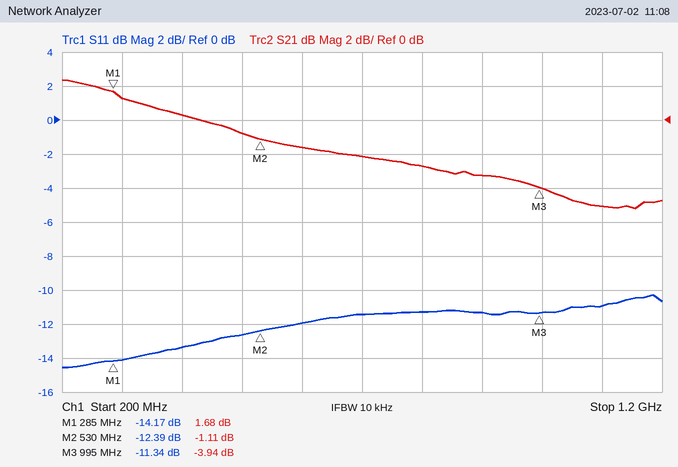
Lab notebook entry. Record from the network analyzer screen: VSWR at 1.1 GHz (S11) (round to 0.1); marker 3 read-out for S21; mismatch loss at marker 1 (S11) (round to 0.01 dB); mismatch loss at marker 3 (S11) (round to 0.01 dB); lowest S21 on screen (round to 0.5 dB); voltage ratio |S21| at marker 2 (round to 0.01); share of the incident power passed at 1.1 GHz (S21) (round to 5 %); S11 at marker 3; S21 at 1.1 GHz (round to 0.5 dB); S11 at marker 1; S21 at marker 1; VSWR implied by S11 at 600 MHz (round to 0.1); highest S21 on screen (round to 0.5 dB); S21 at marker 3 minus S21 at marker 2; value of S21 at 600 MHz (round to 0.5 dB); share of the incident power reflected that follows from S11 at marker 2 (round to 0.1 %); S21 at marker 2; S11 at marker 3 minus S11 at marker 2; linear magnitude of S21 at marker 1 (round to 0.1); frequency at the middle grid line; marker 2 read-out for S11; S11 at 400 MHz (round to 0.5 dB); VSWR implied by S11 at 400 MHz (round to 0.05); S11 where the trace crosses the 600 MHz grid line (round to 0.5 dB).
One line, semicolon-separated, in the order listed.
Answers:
1.8; -3.94 dB; 0.17 dB; 0.33 dB; -5.0 dB; 0.88; 30 %; -11.34 dB; -5.0 dB; -14.17 dB; 1.68 dB; 1.7; 2.5 dB; -2.83 dB; -1.5 dB; 5.8 %; -1.11 dB; 1.05 dB; 1.2; 700 MHz; -12.39 dB; -13.5 dB; 1.55; -12.0 dB
